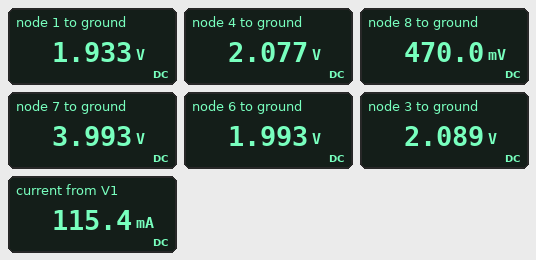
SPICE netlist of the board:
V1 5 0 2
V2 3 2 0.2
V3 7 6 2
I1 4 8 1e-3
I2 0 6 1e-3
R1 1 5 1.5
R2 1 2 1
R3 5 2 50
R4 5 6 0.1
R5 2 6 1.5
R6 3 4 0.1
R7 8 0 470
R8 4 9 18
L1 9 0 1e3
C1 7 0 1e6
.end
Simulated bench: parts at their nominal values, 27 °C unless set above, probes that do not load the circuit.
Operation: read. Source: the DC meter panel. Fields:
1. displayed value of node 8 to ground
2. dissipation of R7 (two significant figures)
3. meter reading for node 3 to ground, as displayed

470.0 mV
470 µW
2.089 V
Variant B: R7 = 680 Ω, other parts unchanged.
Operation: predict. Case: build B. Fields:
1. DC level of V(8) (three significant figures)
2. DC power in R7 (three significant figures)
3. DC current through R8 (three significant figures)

680 mV
680 µW
115 mA
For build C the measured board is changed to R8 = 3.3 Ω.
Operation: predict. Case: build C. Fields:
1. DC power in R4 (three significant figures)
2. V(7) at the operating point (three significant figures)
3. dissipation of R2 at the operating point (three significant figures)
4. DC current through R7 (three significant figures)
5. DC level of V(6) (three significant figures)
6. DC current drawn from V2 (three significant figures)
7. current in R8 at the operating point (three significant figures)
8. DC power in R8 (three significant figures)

9.09 mW
3.97 V
37.5 mW
1.00 mA
1.97 V
506 mA
505 mA
841 mW
